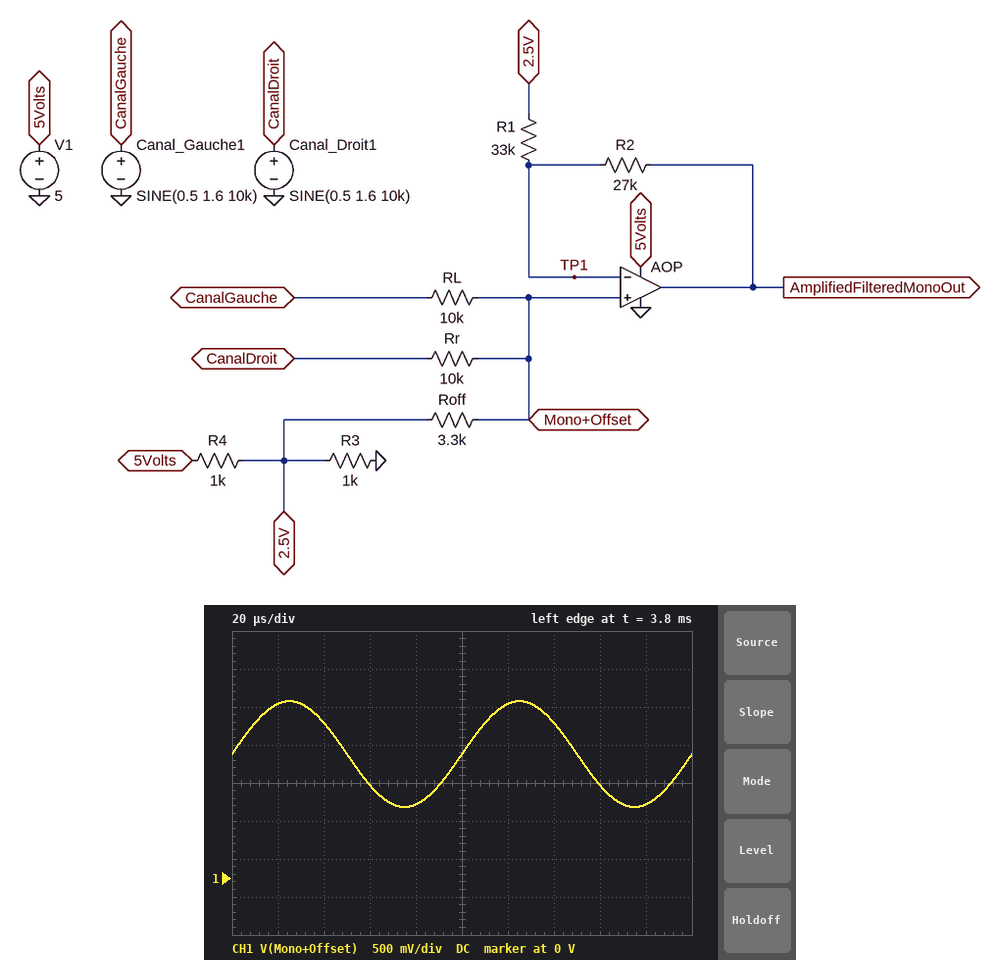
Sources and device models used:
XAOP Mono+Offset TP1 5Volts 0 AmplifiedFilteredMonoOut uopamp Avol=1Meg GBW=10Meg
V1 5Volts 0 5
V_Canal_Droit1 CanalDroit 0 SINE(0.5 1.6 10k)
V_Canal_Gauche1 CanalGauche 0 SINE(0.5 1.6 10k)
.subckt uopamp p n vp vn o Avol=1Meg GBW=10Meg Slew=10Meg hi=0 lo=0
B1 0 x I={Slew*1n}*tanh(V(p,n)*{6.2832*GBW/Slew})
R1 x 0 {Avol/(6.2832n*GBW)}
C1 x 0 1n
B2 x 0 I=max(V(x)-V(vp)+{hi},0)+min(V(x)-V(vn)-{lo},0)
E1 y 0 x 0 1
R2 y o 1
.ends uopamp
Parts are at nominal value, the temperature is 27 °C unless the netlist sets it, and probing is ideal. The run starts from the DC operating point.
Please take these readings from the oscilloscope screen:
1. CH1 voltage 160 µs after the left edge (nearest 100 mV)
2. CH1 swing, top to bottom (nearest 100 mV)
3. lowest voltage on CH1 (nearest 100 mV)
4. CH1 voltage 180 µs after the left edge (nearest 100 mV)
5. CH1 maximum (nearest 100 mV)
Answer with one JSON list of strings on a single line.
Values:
["1.2 V", "1.4 V", "900 mV", "1.0 V", "2.3 V"]
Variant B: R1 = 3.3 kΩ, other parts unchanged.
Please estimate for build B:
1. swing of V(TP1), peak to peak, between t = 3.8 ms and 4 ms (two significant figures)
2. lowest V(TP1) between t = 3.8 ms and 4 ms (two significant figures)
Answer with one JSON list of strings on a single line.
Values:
["300 mV", "2.0 V"]
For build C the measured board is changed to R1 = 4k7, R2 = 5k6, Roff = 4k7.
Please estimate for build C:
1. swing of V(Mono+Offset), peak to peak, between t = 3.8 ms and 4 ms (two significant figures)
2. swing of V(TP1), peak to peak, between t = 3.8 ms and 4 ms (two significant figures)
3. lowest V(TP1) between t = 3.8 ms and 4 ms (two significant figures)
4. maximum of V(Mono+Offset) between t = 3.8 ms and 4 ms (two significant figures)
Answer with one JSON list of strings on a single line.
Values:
["1.7 V", "1.1 V", "1.2 V", "2.3 V"]
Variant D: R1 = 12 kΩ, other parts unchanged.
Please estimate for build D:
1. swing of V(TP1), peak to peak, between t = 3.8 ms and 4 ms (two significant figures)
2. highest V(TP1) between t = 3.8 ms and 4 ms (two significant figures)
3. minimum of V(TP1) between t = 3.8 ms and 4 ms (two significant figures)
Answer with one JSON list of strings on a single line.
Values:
["760 mV", "2.3 V", "1.6 V"]
